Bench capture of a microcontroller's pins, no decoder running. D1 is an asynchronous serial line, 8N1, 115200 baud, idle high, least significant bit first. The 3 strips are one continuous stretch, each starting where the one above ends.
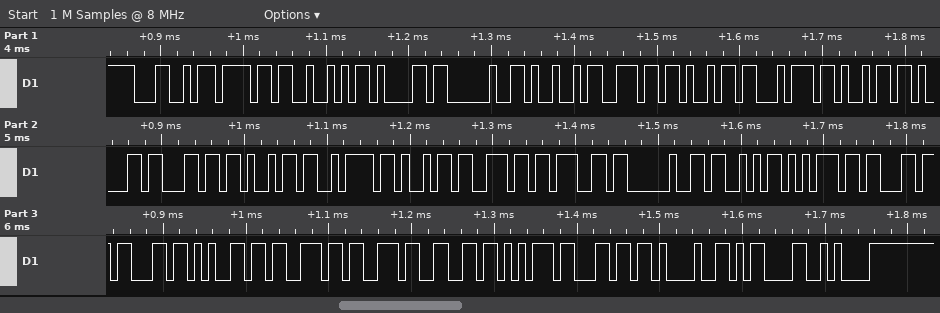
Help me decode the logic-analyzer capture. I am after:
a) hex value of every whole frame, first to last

4C 6F 52 61 20 49 6E 69 74 69 61 6C 69 7A 69 6E 67 20 53 75 63 63 65 73 73 66 75 6C 21 0D 0A
